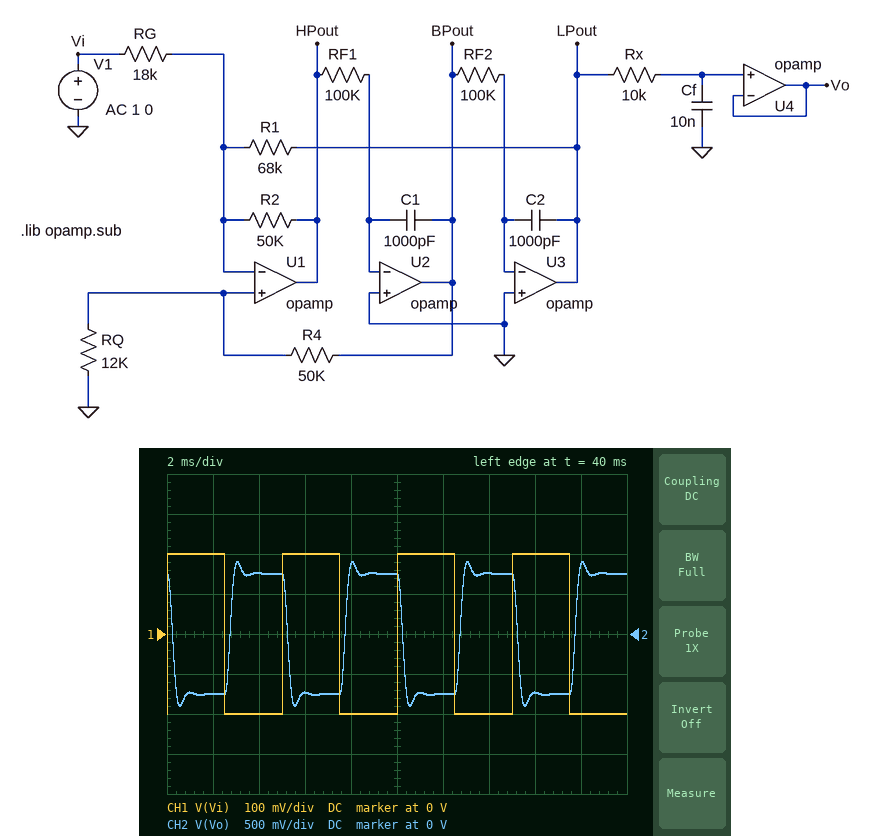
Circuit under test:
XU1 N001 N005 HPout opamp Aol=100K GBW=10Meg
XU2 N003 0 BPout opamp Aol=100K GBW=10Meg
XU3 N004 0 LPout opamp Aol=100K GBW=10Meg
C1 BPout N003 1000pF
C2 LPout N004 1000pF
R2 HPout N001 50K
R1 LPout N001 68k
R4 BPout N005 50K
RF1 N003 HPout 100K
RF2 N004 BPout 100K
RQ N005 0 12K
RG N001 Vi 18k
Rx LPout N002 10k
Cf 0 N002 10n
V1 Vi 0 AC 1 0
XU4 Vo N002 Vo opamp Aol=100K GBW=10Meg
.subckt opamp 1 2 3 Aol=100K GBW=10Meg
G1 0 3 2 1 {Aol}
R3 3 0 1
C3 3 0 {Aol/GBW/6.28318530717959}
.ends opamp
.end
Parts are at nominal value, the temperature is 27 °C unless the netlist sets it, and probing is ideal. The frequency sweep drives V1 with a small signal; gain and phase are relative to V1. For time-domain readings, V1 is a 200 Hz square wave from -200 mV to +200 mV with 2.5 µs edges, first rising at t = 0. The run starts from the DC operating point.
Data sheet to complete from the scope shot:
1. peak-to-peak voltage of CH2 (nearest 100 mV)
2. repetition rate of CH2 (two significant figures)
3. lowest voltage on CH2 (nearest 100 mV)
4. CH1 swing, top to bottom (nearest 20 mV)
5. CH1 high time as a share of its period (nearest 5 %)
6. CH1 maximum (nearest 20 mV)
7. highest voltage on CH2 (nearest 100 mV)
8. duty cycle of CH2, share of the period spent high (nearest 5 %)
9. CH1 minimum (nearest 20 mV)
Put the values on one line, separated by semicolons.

1.8 V; 200 Hz; -900 mV; 400 mV; 50 %; 200 mV; 900 mV; 50 %; -200 mV
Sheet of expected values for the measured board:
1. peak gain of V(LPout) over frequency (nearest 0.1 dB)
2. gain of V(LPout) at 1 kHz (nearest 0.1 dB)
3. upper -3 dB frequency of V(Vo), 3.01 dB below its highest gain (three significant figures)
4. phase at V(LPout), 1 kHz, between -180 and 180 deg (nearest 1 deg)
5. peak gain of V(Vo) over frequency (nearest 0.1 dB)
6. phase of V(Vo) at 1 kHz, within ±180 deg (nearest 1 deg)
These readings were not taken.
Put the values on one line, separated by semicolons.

12.7 dB; 12.7 dB; 1.40 kHz; 122 deg; 11.7 dB; 90 deg
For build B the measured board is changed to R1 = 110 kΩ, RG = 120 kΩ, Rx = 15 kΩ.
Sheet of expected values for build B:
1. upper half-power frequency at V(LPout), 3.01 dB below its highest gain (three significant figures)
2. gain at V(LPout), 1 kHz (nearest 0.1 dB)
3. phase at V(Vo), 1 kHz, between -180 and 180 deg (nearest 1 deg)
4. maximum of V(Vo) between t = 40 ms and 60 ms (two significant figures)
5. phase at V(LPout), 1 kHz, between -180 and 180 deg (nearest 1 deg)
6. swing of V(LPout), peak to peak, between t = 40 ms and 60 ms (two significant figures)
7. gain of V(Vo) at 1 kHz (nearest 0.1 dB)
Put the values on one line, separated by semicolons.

1.26 kHz; 5.0 dB; 61 deg; 280 mV; 105 deg; 680 mV; 2.2 dB
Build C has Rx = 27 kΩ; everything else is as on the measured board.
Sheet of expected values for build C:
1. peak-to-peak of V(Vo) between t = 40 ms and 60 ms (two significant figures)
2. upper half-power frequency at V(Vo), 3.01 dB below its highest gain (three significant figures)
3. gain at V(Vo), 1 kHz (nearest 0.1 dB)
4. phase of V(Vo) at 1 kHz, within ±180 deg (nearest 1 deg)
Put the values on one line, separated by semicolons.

1.5 V; 713 Hz; 6.8 dB; 62 deg
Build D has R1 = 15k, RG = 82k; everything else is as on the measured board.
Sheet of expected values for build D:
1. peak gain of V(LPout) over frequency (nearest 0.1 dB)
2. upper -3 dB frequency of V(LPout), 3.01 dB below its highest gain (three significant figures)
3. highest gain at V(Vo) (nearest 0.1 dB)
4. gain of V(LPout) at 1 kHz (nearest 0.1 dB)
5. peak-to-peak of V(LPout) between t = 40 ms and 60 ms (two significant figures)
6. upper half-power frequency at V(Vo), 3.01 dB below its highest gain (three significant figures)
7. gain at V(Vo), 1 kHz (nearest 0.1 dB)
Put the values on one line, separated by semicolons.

-8.8 dB; 3.40 kHz; -14.5 dB; -13.8 dB; 140 mV; 3.19 kHz; -15.3 dB
